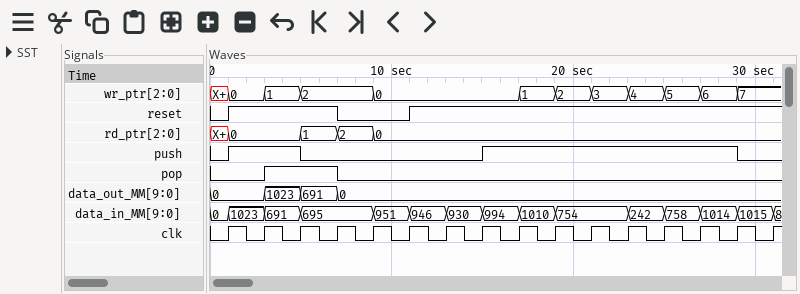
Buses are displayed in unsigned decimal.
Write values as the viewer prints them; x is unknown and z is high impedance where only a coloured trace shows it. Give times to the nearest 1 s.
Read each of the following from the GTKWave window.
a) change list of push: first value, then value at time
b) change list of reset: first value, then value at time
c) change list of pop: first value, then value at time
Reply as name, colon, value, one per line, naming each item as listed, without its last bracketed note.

change list of push: first value, then value at time: 0, 1 at 1 s, 0 at 5 s, 1 at 15 s, 0 at 29 s
change list of reset: first value, then value at time: 0, 1 at 1 s, 0 at 7 s, 1 at 11 s
change list of pop: first value, then value at time: 0, 1 at 3 s, 0 at 7 s
